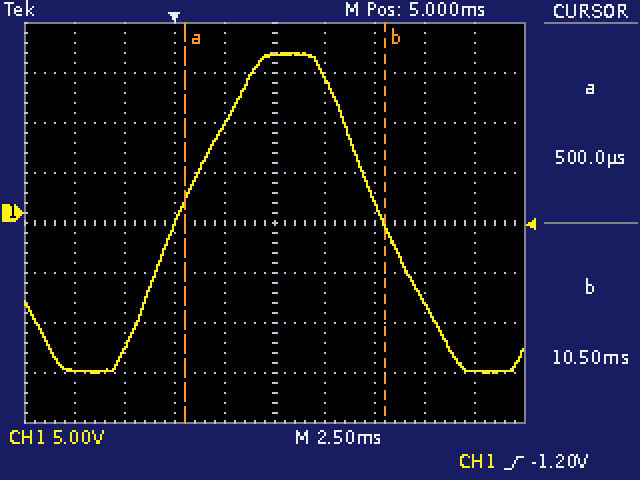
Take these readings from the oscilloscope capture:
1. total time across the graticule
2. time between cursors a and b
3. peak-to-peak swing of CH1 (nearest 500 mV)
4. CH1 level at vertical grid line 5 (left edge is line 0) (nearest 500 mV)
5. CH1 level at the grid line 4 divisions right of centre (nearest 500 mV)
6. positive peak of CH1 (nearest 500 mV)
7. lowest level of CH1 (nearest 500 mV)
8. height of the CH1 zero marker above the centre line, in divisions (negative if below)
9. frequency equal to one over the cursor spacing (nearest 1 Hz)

25 ms
10.00 ms
32.0 V
16.0 V
-16.0 V
16.0 V
-16.0 V
+0.2 div
100 Hz
